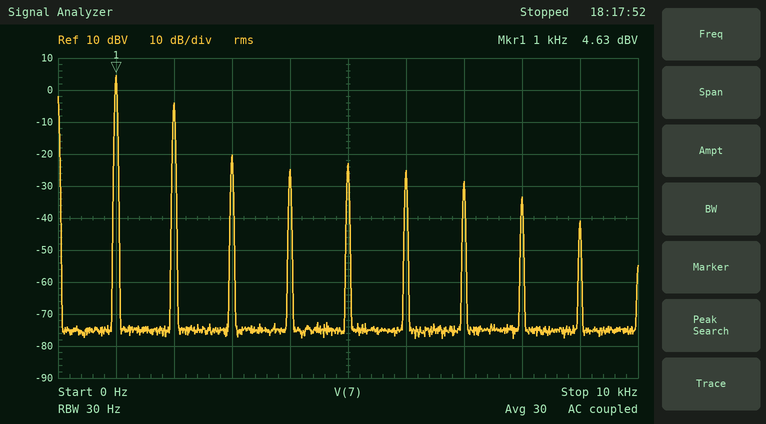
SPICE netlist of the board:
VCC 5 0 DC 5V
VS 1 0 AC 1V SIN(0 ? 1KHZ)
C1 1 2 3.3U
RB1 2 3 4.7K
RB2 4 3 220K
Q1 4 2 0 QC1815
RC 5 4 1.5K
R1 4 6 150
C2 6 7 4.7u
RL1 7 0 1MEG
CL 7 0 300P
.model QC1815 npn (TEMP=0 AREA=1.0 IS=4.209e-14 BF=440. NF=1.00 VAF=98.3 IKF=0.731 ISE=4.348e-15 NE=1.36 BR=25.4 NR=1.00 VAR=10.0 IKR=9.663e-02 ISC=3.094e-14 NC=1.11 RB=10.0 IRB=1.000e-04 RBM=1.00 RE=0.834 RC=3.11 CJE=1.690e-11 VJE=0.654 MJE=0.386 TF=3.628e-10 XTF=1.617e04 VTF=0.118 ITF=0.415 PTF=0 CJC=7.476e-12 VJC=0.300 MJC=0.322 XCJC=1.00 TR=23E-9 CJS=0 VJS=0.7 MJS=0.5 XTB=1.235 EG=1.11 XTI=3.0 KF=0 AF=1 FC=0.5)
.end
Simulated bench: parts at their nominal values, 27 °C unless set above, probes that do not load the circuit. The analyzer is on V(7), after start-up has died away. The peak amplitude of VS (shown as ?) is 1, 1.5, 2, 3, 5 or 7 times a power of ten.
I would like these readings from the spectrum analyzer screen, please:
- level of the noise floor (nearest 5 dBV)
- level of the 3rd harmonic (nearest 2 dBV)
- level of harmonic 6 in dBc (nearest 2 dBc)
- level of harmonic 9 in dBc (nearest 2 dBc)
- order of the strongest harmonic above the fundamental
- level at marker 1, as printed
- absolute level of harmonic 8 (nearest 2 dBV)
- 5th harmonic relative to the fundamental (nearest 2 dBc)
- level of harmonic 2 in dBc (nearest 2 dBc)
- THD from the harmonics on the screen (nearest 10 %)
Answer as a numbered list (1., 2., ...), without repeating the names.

1. -75 dBV
2. -20 dBV
3. -30 dBc
4. -46 dBc
5. 2
6. 4.63 dBV
7. -34 dBV
8. -28 dBc
9. -8 dBc
10. 40 %
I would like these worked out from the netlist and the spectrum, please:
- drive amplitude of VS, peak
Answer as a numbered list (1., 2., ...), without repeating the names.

1. 50 mV
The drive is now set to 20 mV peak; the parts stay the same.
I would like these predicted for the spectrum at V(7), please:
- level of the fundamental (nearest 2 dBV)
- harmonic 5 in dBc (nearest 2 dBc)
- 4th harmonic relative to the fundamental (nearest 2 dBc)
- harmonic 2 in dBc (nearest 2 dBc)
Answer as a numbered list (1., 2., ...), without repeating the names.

1. 2 dBV
2. -38 dBc
3. -38 dBc
4. -16 dBc
